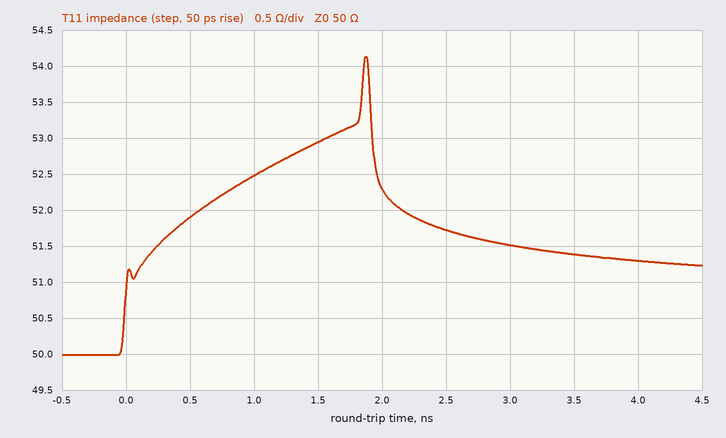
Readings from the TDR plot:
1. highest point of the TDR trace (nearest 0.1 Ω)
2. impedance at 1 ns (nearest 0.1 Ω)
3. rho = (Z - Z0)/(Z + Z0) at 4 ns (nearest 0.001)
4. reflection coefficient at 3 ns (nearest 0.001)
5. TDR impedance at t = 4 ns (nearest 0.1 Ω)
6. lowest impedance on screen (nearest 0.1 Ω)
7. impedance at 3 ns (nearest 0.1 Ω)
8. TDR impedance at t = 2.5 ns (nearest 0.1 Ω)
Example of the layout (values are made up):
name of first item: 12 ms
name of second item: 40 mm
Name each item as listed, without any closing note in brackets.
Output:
highest point of the TDR trace: 54.1 Ω
impedance at 1 ns: 52.5 Ω
rho = (Z - Z0)/(Z + Z0) at 4 ns: +0.013
reflection coefficient at 3 ns: +0.015
TDR impedance at t = 4 ns: 51.3 Ω
lowest impedance on screen: 50.0 Ω
impedance at 3 ns: 51.5 Ω
TDR impedance at t = 2.5 ns: 51.7 Ω
